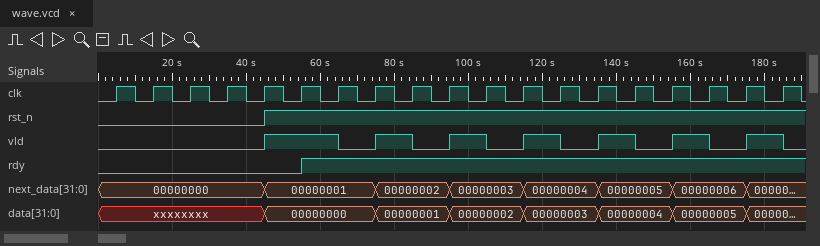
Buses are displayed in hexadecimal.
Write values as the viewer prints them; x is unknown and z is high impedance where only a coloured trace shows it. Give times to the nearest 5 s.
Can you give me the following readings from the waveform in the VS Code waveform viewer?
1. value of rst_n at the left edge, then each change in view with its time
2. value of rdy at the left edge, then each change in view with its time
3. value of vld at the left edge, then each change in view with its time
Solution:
0, 1 at 45 s
0, 1 at 55 s
0, 1 at 45 s, 0 at 65 s, 1 at 75 s, 0 at 85 s, 1 at 95 s, 0 at 105 s, 1 at 115 s, 0 at 125 s, 1 at 135 s, 0 at 145 s, 1 at 155 s, 0 at 165 s, 1 at 175 s, 0 at 185 s
